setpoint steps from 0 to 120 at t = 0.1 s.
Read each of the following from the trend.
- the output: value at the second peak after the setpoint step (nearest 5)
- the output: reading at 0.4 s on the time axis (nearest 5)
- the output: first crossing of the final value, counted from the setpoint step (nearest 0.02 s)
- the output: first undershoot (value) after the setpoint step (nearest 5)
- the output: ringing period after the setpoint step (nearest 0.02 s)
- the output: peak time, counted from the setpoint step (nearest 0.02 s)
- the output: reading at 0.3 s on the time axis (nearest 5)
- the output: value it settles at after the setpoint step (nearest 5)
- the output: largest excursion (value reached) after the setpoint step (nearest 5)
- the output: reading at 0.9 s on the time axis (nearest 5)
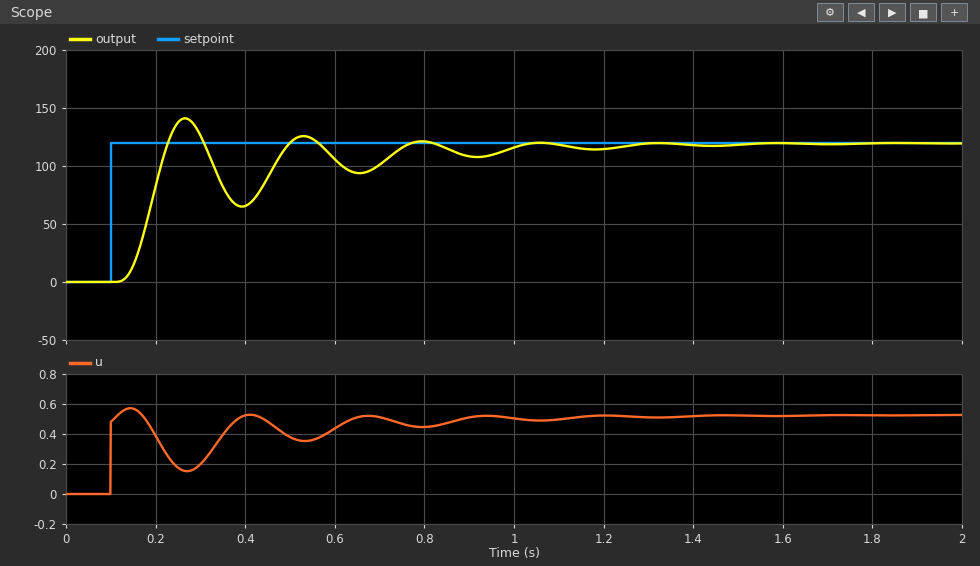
125
65
0.12 s
65
0.26 s
0.16 s
125
120
140
110
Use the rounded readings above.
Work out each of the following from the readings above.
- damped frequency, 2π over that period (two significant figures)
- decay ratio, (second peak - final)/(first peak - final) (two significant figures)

24 rad/s
0.25
